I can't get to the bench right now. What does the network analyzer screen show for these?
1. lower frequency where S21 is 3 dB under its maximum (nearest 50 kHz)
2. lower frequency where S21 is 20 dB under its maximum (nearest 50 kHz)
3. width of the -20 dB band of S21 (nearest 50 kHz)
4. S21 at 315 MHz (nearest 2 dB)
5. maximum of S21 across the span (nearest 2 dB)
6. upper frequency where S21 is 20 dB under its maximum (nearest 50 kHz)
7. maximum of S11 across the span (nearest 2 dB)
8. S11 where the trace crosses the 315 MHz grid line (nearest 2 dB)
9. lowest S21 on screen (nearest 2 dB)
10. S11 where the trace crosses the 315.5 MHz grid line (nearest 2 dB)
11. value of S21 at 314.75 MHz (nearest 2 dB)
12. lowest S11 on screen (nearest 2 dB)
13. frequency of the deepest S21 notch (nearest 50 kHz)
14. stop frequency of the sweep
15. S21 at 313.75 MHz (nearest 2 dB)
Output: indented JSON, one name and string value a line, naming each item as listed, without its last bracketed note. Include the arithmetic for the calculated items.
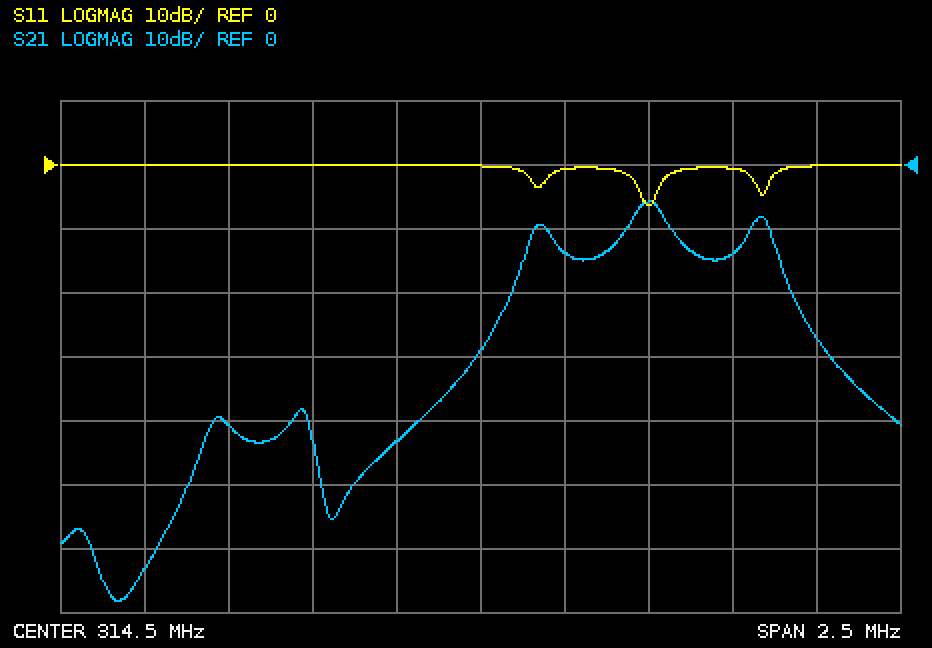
{
  "lower frequency where S21 is 3 dB under its maximum": "314.95 MHz",
  "lower frequency where S21 is 20 dB under its maximum": "314.55 MHz",
  "width of the -20 dB band of S21": "315.50 MHz − 314.55 MHz = 950 kHz",
  "S21 at 315 MHz": "-6 dB",
  "maximum of S21 across the span": "-6 dB",
  "upper frequency where S21 is 20 dB under its maximum": "315.50 MHz",
  "maximum of S11 across the span": "0 dB",
  "S11 where the trace crosses the 315 MHz grid line": "-6 dB",
  "lowest S21 on screen": "-68 dB",
  "S11 where the trace crosses the 315.5 MHz grid line": "0 dB",
  "value of S21 at 314.75 MHz": "-14 dB",
  "lowest S11 on screen": "-6 dB",
  "frequency of the deepest S21 notch": "313.40 MHz",
  "stop frequency of the sweep": "315.75 MHz",
  "S21 at 313.75 MHz": "-40 dB"
}
